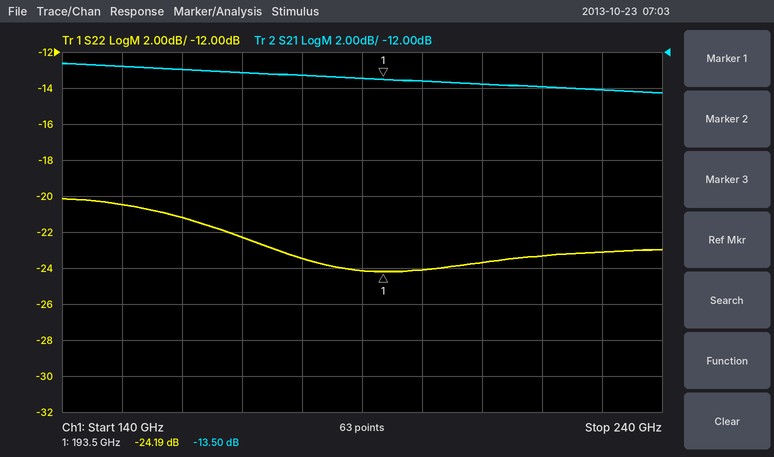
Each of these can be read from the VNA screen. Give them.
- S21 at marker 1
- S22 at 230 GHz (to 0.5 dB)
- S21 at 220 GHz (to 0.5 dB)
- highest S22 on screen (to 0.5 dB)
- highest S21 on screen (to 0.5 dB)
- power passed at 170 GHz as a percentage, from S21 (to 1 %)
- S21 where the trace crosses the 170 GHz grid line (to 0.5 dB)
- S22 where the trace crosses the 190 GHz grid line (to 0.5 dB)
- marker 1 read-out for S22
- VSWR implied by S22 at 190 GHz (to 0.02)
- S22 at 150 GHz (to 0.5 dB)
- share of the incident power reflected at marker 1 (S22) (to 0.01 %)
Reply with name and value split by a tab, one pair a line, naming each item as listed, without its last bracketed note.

S21 at marker 1	-13.50 dB
S22 at 230 GHz	-23.0 dB
S21 at 220 GHz	-14.0 dB
highest S22 on screen	-20.0 dB
highest S21 on screen	-12.5 dB
power passed at 170 GHz as a percentage, from S21	5 %
S21 where the trace crosses the 170 GHz grid line	-13.0 dB
S22 where the trace crosses the 190 GHz grid line	-24.0 dB
marker 1 read-out for S22	-24.19 dB
VSWR implied by S22 at 190 GHz	1.14
S22 at 150 GHz	-20.5 dB
share of the incident power reflected at marker 1 (S22)	0.38 %
